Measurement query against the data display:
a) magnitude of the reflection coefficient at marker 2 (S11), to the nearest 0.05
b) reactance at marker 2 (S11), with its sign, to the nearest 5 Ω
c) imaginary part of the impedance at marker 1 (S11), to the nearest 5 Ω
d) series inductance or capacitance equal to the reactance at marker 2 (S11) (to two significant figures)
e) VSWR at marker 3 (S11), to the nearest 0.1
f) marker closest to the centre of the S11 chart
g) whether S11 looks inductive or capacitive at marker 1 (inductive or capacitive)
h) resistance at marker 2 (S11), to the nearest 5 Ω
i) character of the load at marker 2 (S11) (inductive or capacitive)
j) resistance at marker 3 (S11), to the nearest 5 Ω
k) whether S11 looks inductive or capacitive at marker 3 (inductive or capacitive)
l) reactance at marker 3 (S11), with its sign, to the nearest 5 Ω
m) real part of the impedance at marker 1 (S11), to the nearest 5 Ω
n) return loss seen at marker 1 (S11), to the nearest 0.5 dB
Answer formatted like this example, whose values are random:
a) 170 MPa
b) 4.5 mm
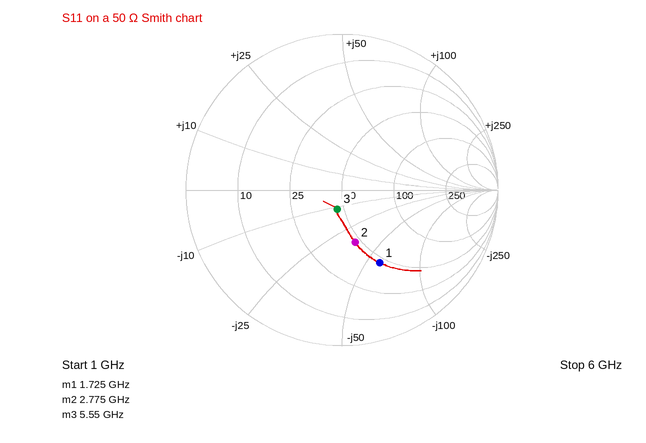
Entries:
a) 0.35
b) -35 Ω
c) -60 Ω
d) 1.6 pF
e) 1.3
f) marker 3
g) capacitive
h) 45 Ω
i) capacitive
j) 45 Ω
k) capacitive
l) -10 Ω
m) 45 Ω
n) 5.5 dB
